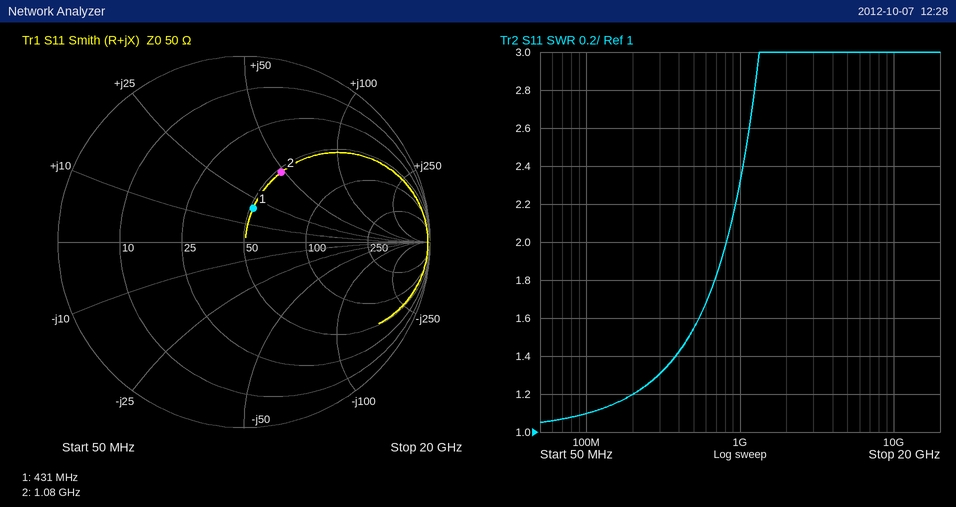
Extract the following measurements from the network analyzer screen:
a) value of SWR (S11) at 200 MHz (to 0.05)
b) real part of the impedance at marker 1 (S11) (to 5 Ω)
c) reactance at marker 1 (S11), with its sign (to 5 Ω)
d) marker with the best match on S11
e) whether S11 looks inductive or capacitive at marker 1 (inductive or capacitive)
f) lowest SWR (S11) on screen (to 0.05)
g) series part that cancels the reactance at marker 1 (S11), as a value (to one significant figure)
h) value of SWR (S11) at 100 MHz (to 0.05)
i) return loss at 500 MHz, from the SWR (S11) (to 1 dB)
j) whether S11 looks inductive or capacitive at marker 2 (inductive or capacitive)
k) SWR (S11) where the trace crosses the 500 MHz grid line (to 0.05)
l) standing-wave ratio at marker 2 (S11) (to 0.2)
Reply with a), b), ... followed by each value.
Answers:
a) 1.20
b) 50 Ω
c) +20 Ω
d) marker 1
e) inductive
f) 1.05
g) 20 pF
h) 1.10
i) 13 dB
j) inductive
k) 1.55
l) 2.4
